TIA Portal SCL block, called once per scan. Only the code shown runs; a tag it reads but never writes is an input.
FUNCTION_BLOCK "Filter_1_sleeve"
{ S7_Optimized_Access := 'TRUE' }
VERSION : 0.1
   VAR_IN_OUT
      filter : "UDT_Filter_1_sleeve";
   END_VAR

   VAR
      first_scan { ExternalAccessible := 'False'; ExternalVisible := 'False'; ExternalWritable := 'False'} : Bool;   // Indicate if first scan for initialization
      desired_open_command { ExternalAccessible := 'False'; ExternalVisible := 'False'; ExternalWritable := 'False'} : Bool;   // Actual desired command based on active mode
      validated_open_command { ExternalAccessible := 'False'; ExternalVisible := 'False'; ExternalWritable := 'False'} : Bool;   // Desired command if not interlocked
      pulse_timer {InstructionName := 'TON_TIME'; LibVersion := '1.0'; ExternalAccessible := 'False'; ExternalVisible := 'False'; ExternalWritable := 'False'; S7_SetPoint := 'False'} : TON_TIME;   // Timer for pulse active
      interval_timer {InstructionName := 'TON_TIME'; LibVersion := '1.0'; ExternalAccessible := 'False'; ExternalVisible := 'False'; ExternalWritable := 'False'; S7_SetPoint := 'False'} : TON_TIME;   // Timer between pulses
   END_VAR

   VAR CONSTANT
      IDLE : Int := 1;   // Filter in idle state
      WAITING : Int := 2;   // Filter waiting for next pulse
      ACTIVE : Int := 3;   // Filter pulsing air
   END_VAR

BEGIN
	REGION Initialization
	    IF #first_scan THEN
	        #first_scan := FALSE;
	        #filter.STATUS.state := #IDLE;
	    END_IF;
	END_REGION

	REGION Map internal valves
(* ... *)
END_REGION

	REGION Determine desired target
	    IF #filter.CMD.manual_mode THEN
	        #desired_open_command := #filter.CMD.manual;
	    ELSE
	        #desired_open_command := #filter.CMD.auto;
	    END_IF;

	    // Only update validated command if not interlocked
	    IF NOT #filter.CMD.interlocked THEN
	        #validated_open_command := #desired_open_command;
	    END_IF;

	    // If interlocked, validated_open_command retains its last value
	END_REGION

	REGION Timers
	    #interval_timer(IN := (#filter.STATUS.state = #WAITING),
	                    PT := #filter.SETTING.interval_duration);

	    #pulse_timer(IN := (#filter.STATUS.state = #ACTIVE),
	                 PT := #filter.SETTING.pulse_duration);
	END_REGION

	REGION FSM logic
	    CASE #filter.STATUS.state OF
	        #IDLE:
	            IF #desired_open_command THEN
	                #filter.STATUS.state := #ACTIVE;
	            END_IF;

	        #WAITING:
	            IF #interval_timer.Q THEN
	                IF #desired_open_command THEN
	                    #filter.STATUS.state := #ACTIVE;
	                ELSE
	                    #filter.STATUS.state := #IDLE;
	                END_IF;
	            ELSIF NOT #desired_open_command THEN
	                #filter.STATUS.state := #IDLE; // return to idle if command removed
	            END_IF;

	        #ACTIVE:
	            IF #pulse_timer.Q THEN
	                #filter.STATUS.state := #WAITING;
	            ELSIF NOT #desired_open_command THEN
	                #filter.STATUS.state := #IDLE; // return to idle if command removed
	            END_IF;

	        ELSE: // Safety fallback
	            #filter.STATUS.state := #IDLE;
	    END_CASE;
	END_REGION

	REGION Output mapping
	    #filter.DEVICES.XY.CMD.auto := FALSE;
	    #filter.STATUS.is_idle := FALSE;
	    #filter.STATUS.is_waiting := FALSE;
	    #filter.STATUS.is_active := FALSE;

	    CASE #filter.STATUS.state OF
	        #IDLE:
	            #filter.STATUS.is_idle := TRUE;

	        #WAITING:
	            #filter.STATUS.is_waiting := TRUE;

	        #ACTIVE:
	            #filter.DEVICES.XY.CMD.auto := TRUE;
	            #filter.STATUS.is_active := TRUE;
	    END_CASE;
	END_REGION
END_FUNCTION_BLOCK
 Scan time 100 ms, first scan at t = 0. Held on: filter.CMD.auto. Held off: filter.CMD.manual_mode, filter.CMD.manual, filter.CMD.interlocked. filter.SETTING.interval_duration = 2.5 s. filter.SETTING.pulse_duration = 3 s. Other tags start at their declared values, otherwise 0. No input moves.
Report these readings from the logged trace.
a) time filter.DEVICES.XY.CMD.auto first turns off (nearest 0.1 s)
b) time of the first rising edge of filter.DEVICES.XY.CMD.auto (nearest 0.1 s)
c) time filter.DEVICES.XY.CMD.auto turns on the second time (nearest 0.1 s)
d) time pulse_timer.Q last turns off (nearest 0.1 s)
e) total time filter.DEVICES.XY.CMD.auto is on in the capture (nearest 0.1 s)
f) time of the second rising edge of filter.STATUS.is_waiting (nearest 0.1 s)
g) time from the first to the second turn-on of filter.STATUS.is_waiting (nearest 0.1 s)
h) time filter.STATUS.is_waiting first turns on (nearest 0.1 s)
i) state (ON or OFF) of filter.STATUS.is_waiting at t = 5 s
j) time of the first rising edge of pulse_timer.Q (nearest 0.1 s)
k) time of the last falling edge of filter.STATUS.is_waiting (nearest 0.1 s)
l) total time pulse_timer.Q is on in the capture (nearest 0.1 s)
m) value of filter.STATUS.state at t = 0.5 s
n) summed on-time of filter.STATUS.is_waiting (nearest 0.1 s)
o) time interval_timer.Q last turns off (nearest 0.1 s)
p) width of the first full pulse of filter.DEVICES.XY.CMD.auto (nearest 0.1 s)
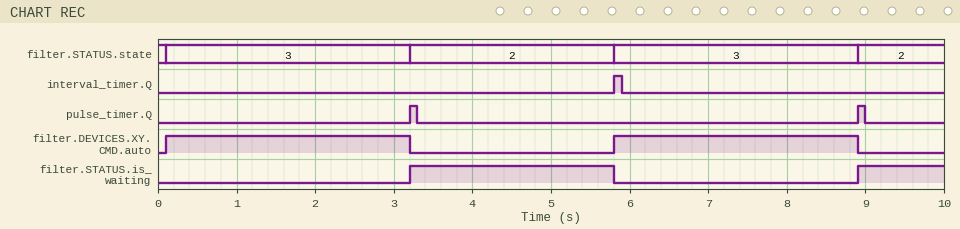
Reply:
3.2 s
0.1 s
5.8 s
9.0 s
6.2 s
8.9 s
5.7 s
3.2 s
ON
3.2 s
5.8 s
0.2 s
3
3.7 s
5.9 s
3.1 s
